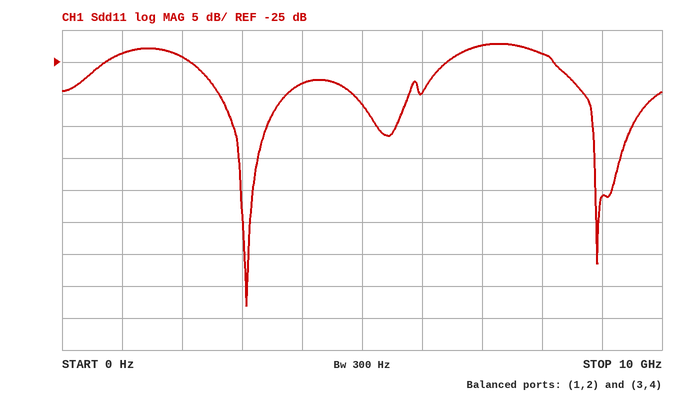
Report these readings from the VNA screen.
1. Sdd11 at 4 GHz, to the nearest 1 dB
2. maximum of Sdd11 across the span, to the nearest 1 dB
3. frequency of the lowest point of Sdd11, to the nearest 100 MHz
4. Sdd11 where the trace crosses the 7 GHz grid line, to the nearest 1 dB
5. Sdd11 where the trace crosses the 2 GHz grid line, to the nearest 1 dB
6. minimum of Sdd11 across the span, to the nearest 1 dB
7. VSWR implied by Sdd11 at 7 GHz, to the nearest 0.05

-28 dB
-22 dB
3.1 GHz
-22 dB
-24 dB
-63 dB
1.15
